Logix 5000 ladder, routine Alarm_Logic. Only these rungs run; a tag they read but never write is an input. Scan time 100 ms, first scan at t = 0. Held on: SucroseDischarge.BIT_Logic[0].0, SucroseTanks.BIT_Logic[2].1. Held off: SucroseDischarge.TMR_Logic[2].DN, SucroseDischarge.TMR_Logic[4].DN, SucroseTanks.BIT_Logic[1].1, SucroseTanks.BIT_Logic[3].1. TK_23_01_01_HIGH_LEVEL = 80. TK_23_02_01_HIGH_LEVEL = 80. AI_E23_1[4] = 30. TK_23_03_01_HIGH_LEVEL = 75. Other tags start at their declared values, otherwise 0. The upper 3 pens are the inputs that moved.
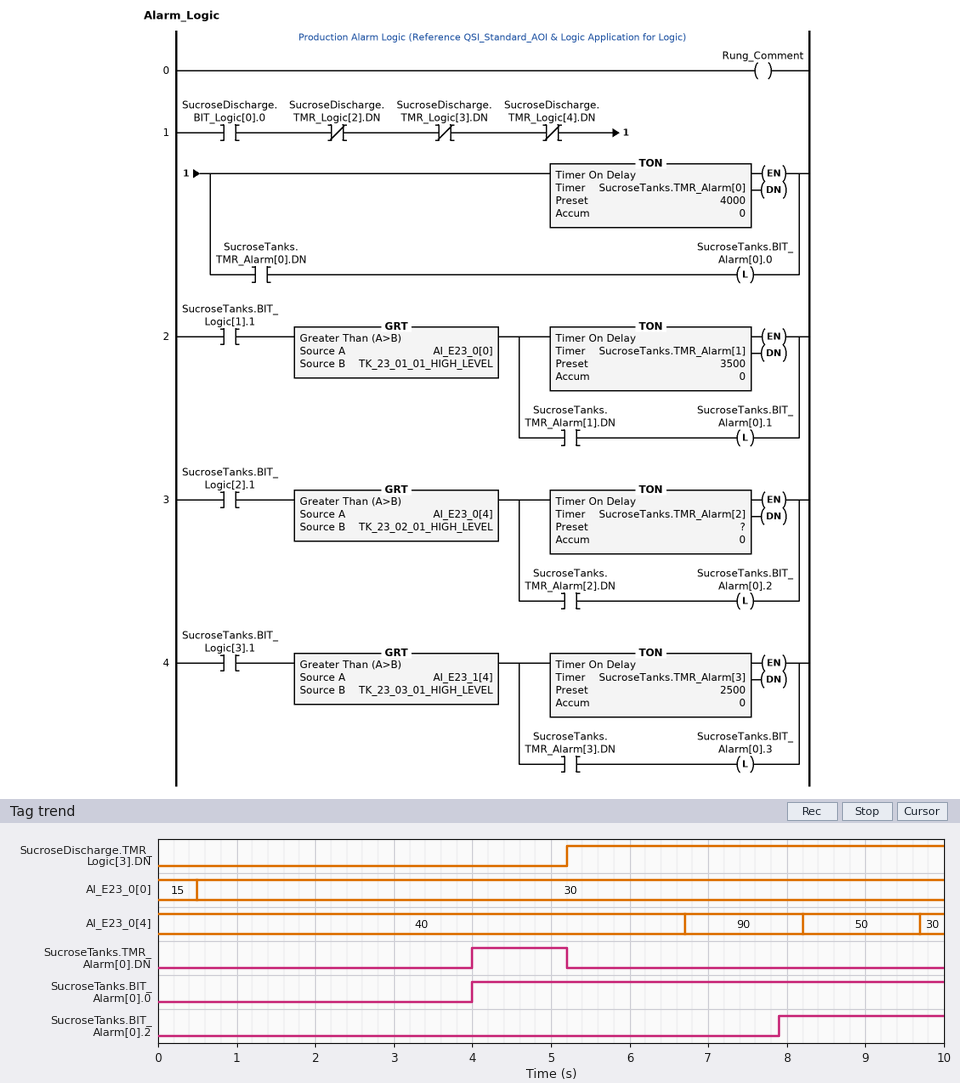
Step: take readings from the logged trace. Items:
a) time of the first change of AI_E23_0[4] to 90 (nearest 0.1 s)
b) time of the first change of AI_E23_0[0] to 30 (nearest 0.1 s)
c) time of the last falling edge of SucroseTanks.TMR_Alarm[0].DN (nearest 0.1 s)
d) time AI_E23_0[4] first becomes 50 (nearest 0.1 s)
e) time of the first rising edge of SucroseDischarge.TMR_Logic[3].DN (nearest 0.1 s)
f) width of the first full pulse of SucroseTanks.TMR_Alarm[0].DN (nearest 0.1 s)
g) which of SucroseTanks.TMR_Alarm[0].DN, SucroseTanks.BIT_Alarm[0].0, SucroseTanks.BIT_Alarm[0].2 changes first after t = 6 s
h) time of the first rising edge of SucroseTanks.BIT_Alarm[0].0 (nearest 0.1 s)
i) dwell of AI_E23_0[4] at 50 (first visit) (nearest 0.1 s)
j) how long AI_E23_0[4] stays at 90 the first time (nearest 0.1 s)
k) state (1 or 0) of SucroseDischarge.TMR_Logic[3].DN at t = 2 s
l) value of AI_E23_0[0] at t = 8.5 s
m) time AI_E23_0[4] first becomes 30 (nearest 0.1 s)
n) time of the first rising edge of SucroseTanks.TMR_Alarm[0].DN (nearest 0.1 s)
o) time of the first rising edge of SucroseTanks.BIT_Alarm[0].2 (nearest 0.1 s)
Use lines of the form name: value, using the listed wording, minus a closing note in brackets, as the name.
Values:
time of the first change of AI_E23_0[4] to 90: 6.7 s
time of the first change of AI_E23_0[0] to 30: 0.5 s
time of the last falling edge of SucroseTanks.TMR_Alarm[0].DN: 5.2 s
time AI_E23_0[4] first becomes 50: 8.2 s
time of the first rising edge of SucroseDischarge.TMR_Logic[3].DN: 5.2 s
width of the first full pulse of SucroseTanks.TMR_Alarm[0].DN: 1.2 s
which of SucroseTanks.TMR_Alarm[0].DN, SucroseTanks.BIT_Alarm[0].0, SucroseTanks.BIT_Alarm[0].2 changes first after t = 6 s: SucroseTanks.BIT_Alarm[0].2
time of the first rising edge of SucroseTanks.BIT_Alarm[0].0: 4.0 s
dwell of AI_E23_0[4] at 50 (first visit): 1.5 s
how long AI_E23_0[4] stays at 90 the first time: 1.5 s
state (1 or 0) of SucroseDischarge.TMR_Logic[3].DN at t = 2 s: 0
value of AI_E23_0[0] at t = 8.5 s: 30
time AI_E23_0[4] first becomes 30: 9.7 s
time of the first rising edge of SucroseTanks.TMR_Alarm[0].DN: 4.0 s
time of the first rising edge of SucroseTanks.BIT_Alarm[0].2: 7.9 s
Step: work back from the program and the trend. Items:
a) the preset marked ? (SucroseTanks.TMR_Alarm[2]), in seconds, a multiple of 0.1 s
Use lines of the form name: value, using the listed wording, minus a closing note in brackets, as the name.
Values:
the preset marked ? (SucroseTanks.TMR_Alarm[2]), in seconds, a multiple of 0.1 s: 1.2 s
